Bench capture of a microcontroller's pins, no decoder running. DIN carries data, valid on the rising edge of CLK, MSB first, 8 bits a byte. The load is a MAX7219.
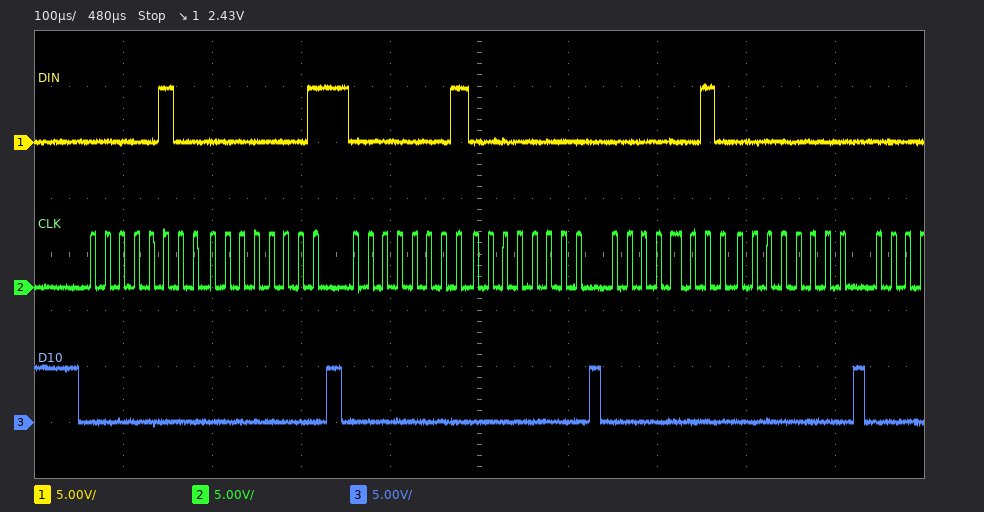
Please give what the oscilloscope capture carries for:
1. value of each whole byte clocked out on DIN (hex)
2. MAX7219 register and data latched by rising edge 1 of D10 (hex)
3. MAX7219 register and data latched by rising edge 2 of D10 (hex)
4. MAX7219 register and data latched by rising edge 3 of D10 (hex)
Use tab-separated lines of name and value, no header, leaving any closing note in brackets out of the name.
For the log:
value of each whole byte clocked out on DIN	04 01 01 00 02 00
MAX7219 register and data latched by rising edge 1 of D10	register 0x4, data 0x01
MAX7219 register and data latched by rising edge 2 of D10	register 0x1, data 0x00
MAX7219 register and data latched by rising edge 3 of D10	register 0x2, data 0x00
